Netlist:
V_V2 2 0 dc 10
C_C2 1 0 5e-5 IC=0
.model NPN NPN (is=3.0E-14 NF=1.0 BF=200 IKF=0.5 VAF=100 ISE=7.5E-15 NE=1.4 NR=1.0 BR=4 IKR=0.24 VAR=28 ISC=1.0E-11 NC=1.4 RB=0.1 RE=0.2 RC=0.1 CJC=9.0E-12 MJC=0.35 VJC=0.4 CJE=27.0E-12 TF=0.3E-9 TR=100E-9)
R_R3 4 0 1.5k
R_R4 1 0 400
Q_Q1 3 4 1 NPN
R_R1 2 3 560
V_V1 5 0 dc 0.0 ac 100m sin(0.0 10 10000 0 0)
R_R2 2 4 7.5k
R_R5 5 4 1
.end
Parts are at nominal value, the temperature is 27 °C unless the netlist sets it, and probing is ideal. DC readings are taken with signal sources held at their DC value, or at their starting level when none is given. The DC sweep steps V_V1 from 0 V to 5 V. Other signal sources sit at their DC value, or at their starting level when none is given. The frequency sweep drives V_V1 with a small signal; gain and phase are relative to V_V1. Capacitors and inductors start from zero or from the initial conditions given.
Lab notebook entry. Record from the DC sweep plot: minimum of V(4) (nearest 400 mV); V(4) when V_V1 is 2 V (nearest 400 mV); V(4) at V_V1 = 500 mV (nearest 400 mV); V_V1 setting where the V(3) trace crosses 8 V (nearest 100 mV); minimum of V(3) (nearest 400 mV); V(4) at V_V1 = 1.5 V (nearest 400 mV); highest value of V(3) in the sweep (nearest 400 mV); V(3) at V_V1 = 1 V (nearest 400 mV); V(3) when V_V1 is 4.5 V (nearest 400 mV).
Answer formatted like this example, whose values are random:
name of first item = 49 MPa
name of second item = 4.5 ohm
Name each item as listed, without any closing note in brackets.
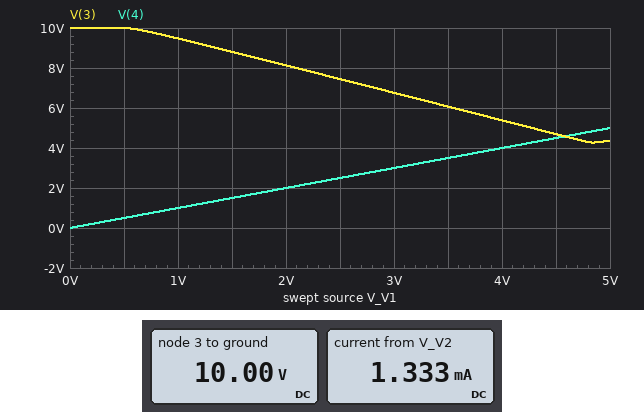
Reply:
minimum of V(4) = 0 V
V(4) when V_V1 is 2 V = 2.0 V
V(4) at V_V1 = 500 mV = 400 mV
V_V1 setting where the V(3) trace crosses 8 V = 2.1 V
minimum of V(3) = 4.4 V
V(4) at V_V1 = 1.5 V = 1.6 V
highest value of V(3) in the sweep = 10.0 V
V(3) at V_V1 = 1 V = 9.6 V
V(3) when V_V1 is 4.5 V = 4.8 V
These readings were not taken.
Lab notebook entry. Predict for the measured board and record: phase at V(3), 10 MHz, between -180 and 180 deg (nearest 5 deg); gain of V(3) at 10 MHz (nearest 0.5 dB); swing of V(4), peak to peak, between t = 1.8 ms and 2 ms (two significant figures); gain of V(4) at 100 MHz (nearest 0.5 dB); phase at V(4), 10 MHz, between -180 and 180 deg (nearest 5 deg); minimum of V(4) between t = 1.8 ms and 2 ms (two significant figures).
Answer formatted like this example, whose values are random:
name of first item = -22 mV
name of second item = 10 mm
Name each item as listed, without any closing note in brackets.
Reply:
phase at V(3), 10 MHz, between -180 and 180 deg = 85 deg
gain of V(3) at 10 MHz = -20.0 dB
swing of V(4), peak to peak, between t = 1.8 ms and 2 ms = 20 V
gain of V(4) at 100 MHz = 0 dB
phase at V(4), 10 MHz, between -180 and 180 deg = 0 deg
minimum of V(4) between t = 1.8 ms and 2 ms = -10 V
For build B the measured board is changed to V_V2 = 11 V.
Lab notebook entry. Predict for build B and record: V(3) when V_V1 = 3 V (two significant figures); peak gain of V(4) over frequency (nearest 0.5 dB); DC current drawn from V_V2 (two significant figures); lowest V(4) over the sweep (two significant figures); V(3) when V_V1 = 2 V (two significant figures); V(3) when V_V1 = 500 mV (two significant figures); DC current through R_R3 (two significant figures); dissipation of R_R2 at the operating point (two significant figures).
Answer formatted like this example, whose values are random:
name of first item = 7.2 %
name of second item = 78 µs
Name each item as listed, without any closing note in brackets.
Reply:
V(3) when V_V1 = 3 V = 7.8 V
peak gain of V(4) over frequency = 0 dB
DC current drawn from V_V2 = 1.5 mA
lowest V(4) over the sweep = 1.5 mV
V(3) when V_V1 = 2 V = 9.1 V
V(3) when V_V1 = 500 mV = 11 V
DC current through R_R3 = 980 nA
dissipation of R_R2 at the operating point = 16 mW
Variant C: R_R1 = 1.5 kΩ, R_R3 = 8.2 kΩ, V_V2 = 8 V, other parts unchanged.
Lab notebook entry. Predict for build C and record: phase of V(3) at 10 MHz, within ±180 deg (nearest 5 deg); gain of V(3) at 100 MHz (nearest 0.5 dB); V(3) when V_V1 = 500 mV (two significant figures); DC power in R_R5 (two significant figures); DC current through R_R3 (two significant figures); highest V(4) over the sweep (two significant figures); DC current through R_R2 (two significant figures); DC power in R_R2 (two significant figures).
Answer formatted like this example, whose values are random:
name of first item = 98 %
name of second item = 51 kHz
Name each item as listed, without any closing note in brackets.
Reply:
phase of V(3) at 10 MHz, within ±180 deg = 75 deg
gain of V(3) at 100 MHz = -0.5 dB
V(3) when V_V1 = 500 mV = 8.0 V
DC power in R_R5 = 1.1 µW
DC current through R_R3 = 130 nA
highest V(4) over the sweep = 5.0 V
DC current through R_R2 = 1.1 mA
DC power in R_R2 = 8.5 mW
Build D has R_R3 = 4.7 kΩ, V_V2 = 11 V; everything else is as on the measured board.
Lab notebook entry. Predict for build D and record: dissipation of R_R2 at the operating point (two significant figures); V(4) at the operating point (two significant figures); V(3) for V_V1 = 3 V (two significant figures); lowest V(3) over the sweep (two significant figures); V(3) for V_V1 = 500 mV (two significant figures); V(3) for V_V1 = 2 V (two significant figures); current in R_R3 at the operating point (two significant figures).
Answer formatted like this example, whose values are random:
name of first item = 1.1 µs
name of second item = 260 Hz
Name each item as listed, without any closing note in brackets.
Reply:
dissipation of R_R2 at the operating point = 16 mW
V(4) at the operating point = 1.5 mV
V(3) for V_V1 = 3 V = 7.8 V
lowest V(3) over the sweep = 5.0 V
V(3) for V_V1 = 500 mV = 11 V
V(3) for V_V1 = 2 V = 9.1 V
current in R_R3 at the operating point = 310 nA
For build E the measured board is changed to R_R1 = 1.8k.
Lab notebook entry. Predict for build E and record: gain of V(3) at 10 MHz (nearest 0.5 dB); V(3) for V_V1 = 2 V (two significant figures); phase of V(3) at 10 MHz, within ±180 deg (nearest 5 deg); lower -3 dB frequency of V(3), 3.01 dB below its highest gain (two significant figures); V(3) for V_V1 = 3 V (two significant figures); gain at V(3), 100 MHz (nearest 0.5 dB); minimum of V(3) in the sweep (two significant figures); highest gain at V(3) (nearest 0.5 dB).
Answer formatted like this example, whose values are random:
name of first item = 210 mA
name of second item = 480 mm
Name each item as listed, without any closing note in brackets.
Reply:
gain of V(3) at 10 MHz = -10.0 dB
V(3) for V_V1 = 2 V = 4.0 V
phase of V(3) at 10 MHz, within ±180 deg = 70 deg
lower -3 dB frequency of V(3), 3.01 dB below its highest gain = 30 MHz
V(3) for V_V1 = 3 V = 2.3 V
gain at V(3), 100 MHz = -0.5 dB
minimum of V(3) in the sweep = 1.9 V
highest gain at V(3) = 0 dB
